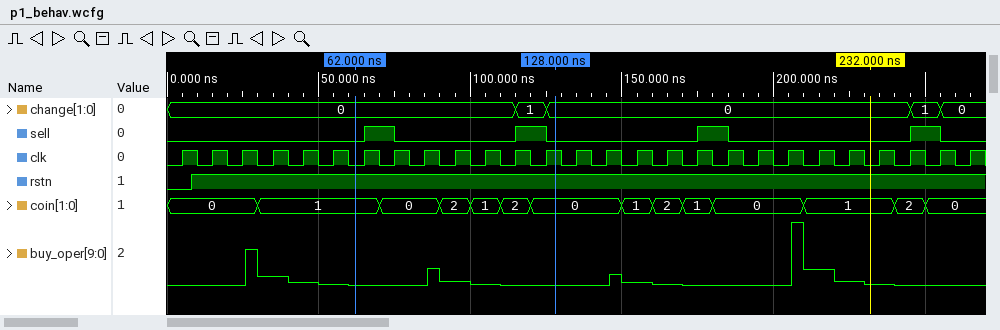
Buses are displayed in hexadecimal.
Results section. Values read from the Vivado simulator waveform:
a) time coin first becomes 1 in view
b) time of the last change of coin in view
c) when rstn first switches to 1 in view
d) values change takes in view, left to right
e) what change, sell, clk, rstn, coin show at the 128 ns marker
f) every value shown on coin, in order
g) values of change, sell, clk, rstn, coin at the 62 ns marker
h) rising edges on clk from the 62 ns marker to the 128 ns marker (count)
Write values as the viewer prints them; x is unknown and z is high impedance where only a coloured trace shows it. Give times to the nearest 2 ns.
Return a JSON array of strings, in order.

["30 ns", "250 ns", "8 ns", "0, 1, 0, 1, 0", "change=0, sell=0, clk=1, rstn=1, coin=0", "0, 1, 0, 2, 1, 2, 0, 1, 2, 1, 0, 1, 2, 0", "change=0, sell=0, clk=0, rstn=1, coin=1", "7"]
